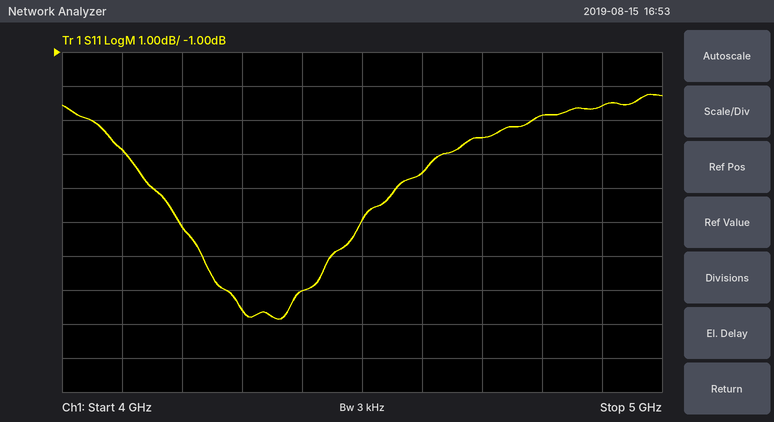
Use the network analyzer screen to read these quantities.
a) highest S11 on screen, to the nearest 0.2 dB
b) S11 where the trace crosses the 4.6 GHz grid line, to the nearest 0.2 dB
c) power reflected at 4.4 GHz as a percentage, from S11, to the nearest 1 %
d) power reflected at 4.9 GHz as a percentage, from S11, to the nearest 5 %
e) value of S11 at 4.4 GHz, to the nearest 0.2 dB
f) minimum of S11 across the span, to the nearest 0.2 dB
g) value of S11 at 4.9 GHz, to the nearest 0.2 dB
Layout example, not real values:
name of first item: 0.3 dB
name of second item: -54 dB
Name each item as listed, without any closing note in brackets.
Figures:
highest S11 on screen, to the nearest 0.2 dB: -2.2 dB
S11 where the trace crosses the 4.6 GHz grid line, to the nearest 0.2 dB: -4.6 dB
power reflected at 4.4 GHz as a percentage, from S11, to the nearest 1 %: 16 %
power reflected at 4.9 GHz as a percentage, from S11, to the nearest 5 %: 55 %
value of S11 at 4.4 GHz, to the nearest 0.2 dB: -8.0 dB
minimum of S11 across the span, to the nearest 0.2 dB: -8.8 dB
value of S11 at 4.9 GHz, to the nearest 0.2 dB: -2.6 dB
